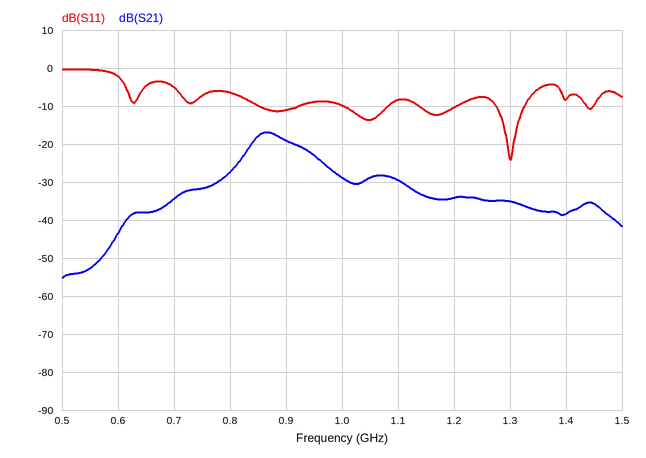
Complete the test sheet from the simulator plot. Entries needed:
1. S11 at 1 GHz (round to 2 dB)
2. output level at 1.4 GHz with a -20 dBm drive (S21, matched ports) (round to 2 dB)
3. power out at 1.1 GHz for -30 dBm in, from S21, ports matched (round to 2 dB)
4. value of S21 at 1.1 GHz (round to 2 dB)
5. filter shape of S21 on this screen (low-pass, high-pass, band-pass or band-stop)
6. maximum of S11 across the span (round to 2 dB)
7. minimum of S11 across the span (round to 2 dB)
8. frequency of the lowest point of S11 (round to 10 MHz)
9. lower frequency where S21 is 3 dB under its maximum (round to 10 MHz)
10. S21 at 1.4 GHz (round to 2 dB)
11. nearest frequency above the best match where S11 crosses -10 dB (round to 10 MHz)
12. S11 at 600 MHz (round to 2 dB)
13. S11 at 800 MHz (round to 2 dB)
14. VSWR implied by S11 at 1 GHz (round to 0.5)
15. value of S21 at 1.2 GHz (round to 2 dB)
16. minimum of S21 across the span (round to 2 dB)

-10 dB
-58 dBm
-60 dBm
-30 dB
band-pass
0 dB
-24 dB
1.30 GHz
840 MHz
-38 dB
1.33 GHz
-2 dB
-6 dB
2.0
-34 dB
-56 dB
